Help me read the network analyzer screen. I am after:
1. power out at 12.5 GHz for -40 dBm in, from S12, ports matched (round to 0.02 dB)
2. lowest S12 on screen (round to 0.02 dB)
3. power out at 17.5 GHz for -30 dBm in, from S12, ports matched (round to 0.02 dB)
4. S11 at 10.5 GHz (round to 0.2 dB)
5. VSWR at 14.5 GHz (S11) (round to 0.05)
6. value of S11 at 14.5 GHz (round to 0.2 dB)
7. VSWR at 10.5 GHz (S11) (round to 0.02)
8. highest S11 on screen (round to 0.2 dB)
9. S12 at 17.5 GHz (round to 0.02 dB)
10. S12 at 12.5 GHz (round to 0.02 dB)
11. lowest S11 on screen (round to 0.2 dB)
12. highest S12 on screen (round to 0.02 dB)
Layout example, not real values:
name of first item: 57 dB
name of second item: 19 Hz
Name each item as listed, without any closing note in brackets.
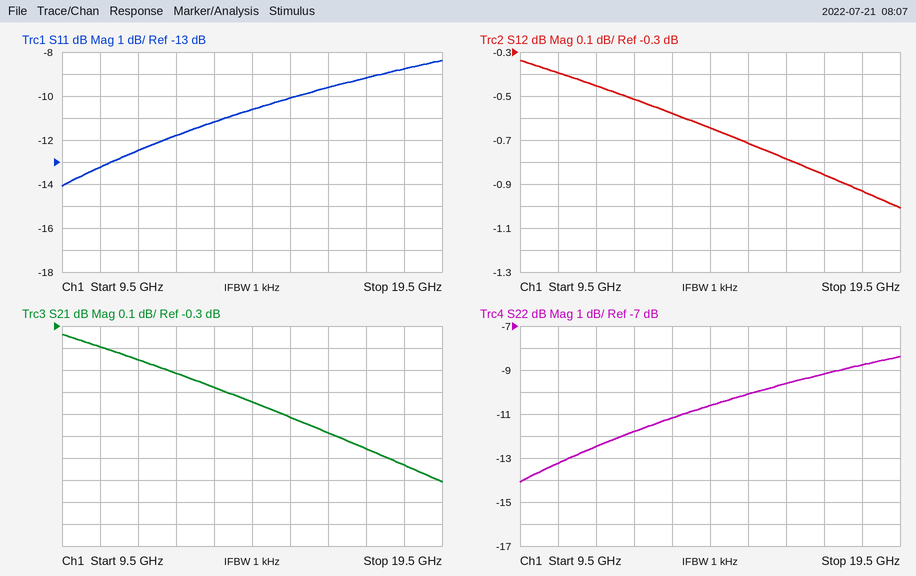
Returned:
power out at 12.5 GHz for -40 dBm in, from S12, ports matched: -40.52 dBm
lowest S12 on screen: -1.00 dB
power out at 17.5 GHz for -30 dBm in, from S12, ports matched: -30.86 dBm
S11 at 10.5 GHz: -13.2 dB
VSWR at 14.5 GHz (S11): 1.85
value of S11 at 14.5 GHz: -10.6 dB
VSWR at 10.5 GHz (S11): 1.56
highest S11 on screen: -8.4 dB
S12 at 17.5 GHz: -0.86 dB
S12 at 12.5 GHz: -0.52 dB
lowest S11 on screen: -14.0 dB
highest S12 on screen: -0.34 dB
